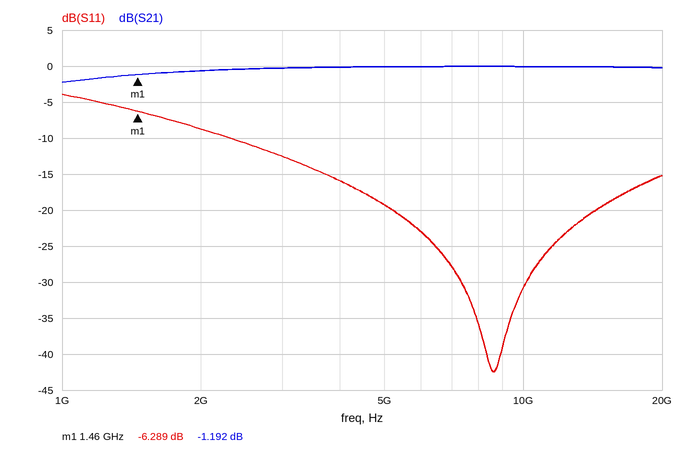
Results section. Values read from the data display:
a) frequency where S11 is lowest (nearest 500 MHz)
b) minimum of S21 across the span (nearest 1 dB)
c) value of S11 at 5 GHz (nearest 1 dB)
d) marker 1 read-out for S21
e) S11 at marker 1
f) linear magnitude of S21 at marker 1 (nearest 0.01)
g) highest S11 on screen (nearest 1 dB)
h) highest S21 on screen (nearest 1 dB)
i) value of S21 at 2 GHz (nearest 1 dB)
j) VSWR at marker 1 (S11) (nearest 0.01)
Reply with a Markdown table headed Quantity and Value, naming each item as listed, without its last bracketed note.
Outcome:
| Quantity | Value |
|---|---|
| frequency where S11 is lowest | 8.5 GHz |
| minimum of S21 across the span | -2 dB |
| value of S11 at 5 GHz | -19 dB |
| marker 1 read-out for S21 | -1.192 dB |
| S11 at marker 1 | -6.289 dB |
| linear magnitude of S21 at marker 1 | 0.87 |
| highest S11 on screen | -4 dB |
| highest S21 on screen | 0 dB |
| value of S21 at 2 GHz | -1 dB |
| VSWR at marker 1 (S11) | 2.88 |
